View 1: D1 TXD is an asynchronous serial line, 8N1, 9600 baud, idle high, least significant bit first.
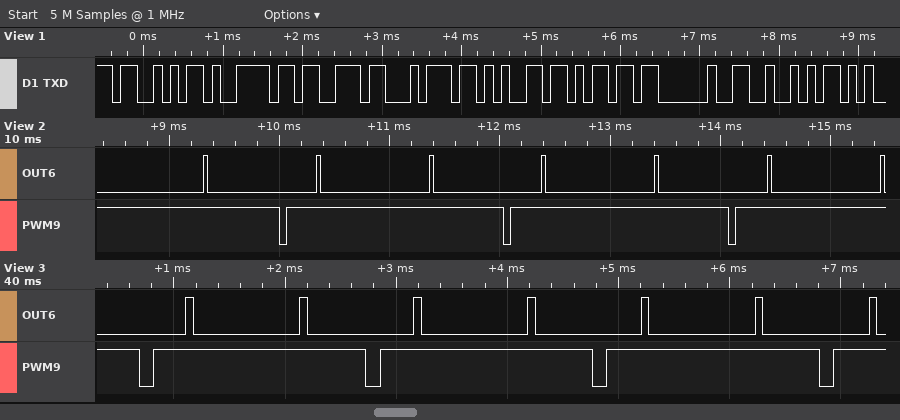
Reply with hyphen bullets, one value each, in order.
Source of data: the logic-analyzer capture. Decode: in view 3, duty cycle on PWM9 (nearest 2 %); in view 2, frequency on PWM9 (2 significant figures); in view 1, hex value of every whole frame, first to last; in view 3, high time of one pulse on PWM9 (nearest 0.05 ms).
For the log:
- 94 %
- 490 Hz
- 53 79 73 74 65 6D 20 52
- 1.90 ms
